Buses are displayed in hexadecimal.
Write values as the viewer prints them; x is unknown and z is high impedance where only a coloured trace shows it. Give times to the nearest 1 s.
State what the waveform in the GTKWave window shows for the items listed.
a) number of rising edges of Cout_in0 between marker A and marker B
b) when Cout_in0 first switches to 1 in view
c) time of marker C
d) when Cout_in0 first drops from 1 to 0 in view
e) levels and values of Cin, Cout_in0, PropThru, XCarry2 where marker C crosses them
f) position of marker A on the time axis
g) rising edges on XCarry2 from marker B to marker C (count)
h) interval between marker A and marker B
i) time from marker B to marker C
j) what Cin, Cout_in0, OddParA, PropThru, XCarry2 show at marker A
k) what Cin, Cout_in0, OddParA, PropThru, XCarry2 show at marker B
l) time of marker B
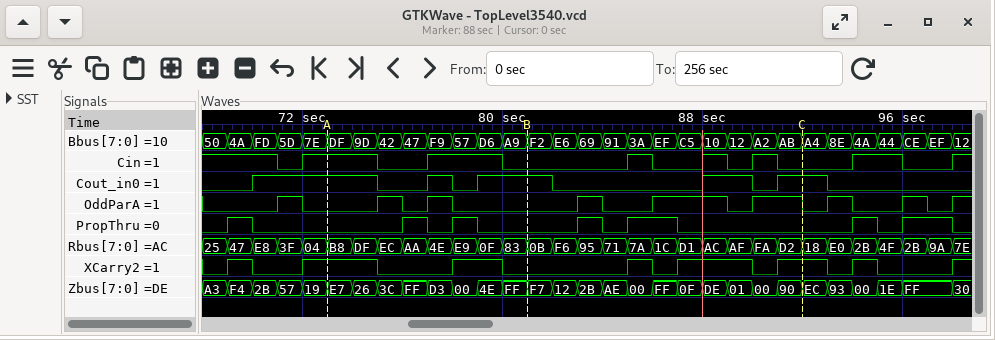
2
70 s
92 s
75 s
Cin=0, Cout_in0=1, PropThru=0, XCarry2=1
73 s
3
8 s
11 s
Cin=1, Cout_in0=1, OddParA=0, PropThru=0, XCarry2=1
Cin=0, Cout_in0=1, OddParA=0, PropThru=0, XCarry2=0
81 s
